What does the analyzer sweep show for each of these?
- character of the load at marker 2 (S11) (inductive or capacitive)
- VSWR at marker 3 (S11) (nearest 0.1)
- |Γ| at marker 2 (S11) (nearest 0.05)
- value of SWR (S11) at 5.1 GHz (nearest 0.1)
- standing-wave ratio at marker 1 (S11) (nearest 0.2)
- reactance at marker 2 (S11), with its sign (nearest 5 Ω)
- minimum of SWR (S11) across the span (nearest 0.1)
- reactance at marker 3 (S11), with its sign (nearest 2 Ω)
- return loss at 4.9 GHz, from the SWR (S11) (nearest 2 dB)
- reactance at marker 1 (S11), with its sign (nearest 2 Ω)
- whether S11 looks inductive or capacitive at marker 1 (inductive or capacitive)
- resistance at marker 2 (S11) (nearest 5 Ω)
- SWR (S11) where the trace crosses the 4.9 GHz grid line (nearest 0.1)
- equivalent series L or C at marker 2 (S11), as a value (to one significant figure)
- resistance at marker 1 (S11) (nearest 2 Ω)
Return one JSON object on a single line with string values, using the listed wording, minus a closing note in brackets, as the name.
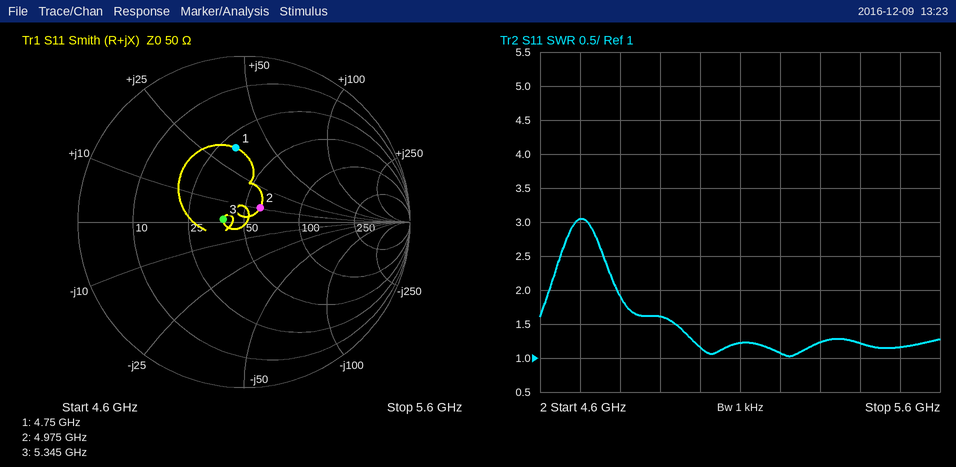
{"character of the load at marker 2 (S11)": "inductive", "VSWR at marker 3 (S11)": "1.3", "|Γ| at marker 2 (S11)": "0.15", "value of SWR (S11) at 5.1 GHz": "1.2", "standing-wave ratio at marker 1 (S11)": "2.6", "reactance at marker 2 (S11), with its sign": "+10 Ω", "minimum of SWR (S11) across the span": "1.0", "reactance at marker 3 (S11), with its sign": "+2 Ω", "return loss at 4.9 GHz, from the SWR (S11)": "12 dB", "reactance at marker 1 (S11), with its sign": "+34 Ω", "whether S11 looks inductive or capacitive at marker 1": "inductive", "resistance at marker 2 (S11)": "60 Ω", "SWR (S11) where the trace crosses the 4.9 GHz grid line": "1.6", "equivalent series L or C at marker 2 (S11), as a value": "300 pH", "resistance at marker 1 (S11)": "30 Ω"}
